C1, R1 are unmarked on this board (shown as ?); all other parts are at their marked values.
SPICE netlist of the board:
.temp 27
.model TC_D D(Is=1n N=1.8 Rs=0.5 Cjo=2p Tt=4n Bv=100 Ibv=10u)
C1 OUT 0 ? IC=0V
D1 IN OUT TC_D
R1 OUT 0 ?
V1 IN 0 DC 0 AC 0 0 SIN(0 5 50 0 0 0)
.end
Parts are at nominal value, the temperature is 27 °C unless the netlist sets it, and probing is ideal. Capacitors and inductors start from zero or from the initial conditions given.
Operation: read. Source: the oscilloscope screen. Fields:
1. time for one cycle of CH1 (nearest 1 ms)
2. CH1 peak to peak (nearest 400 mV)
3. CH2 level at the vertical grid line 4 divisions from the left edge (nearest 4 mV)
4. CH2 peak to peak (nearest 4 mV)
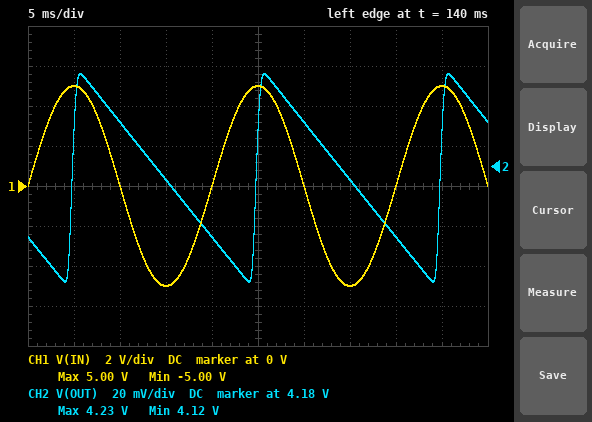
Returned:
20 ms
10.0 V
4.144 V
104 mV
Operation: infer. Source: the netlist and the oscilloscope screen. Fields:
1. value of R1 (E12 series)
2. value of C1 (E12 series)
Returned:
3.3 kΩ
220 µF
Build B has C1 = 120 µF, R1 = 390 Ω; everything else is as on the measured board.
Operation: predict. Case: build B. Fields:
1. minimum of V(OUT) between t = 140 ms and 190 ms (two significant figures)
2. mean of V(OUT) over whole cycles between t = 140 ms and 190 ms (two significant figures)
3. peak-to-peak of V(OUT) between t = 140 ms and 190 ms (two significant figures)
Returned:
2.9 V
3.6 V
1.3 V
